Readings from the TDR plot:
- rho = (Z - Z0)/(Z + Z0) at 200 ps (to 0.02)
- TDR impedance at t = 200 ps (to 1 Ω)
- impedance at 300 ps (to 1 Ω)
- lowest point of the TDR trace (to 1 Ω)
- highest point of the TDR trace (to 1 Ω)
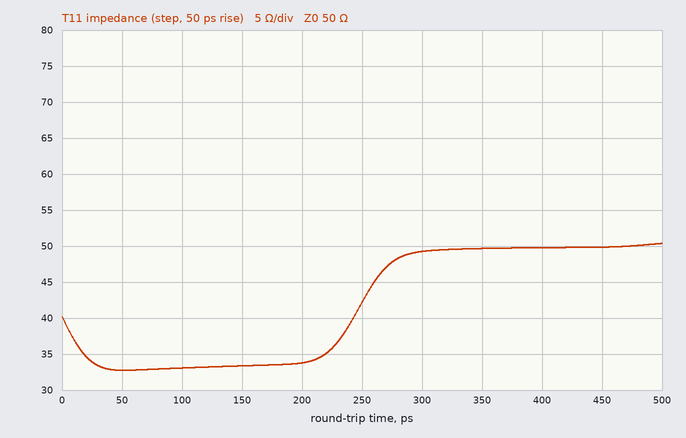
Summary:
-0.20
34 Ω
49 Ω
33 Ω
50 Ω
